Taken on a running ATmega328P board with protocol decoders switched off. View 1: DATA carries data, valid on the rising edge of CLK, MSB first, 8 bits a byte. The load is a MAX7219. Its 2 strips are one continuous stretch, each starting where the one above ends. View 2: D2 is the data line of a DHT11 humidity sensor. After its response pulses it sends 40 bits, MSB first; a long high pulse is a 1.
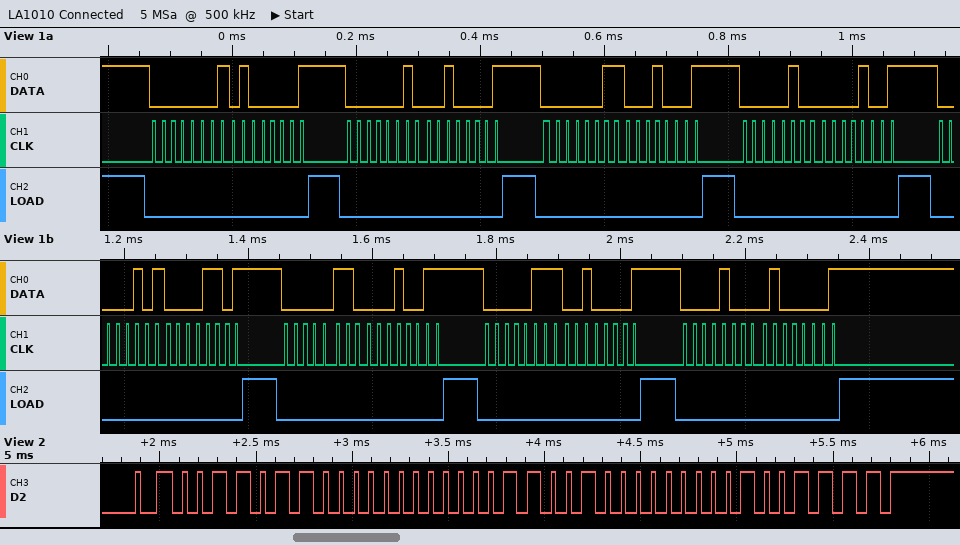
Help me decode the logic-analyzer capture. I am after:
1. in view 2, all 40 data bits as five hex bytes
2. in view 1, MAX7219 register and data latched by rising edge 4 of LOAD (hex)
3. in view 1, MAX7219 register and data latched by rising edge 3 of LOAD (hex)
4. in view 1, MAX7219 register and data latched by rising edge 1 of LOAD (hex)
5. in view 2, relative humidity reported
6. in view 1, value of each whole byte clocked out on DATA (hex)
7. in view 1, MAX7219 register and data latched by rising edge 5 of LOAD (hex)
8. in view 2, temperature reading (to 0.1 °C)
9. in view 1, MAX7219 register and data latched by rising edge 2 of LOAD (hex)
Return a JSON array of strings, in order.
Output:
["36 00 19 00 4F", "register 0x4, data 0x09", "register 0x3, data 0x11", "register 0x1, data 0x41", "54 %", "0x01 0x41 0x02 0x21 0x03 0x11 0x04 0x09 0x05 0x0D 0x06 0x13 0x07 0x21 0x08 0x41", "register 0x5, data 0x0D", "25.0 °C", "register 0x2, data 0x21"]
